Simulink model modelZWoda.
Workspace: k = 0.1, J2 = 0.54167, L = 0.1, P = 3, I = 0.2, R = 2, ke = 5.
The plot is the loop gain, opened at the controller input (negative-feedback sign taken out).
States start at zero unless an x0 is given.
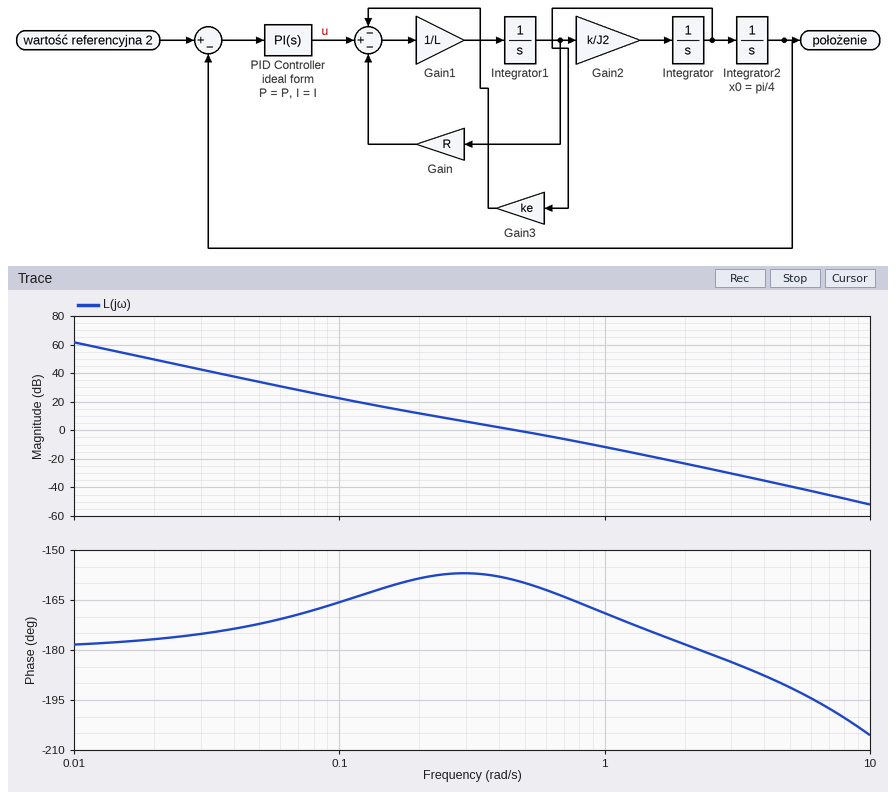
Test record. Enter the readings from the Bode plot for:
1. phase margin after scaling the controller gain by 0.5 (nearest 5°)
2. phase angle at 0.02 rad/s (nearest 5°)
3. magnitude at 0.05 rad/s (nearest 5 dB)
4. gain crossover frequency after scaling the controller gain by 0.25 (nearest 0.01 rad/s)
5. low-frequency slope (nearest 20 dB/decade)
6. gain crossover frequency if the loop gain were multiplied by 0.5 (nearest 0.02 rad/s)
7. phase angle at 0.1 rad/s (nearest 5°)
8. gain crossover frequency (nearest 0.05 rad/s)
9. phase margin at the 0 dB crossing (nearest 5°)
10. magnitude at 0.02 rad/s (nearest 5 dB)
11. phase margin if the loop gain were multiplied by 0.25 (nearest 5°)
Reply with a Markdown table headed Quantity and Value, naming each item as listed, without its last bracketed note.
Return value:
| Quantity | Value |
|---|---|
| phase margin after scaling the controller gain by 0.5 | 25° |
| phase angle at 0.02 rad/s | -175° |
| magnitude at 0.05 rad/s | 35 dB |
| gain crossover frequency after scaling the controller gain by 0.25 | 0.20 rad/s |
| low-frequency slope | -40 dB/decade |
| gain crossover frequency if the loop gain were multiplied by 0.5 | 0.30 rad/s |
| phase angle at 0.1 rad/s | -165° |
| gain crossover frequency | 0.45 rad/s |
| phase margin at the 0 dB crossing | 20° |
| magnitude at 0.02 rad/s | 50 dB |
| phase margin if the loop gain were multiplied by 0.25 | 20° |
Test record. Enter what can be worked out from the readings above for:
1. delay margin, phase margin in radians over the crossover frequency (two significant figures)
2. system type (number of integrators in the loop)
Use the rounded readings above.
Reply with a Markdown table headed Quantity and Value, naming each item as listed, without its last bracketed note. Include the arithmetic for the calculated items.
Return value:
| Quantity | Value |
|---|---|
| delay margin, phase margin in radians over the crossover frequency | 20 × π / 180 / 0.45 = 0.78 s |
| system type | 2 |
